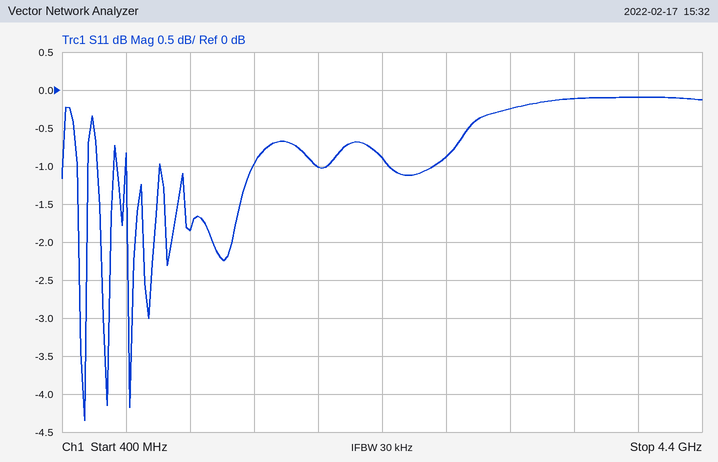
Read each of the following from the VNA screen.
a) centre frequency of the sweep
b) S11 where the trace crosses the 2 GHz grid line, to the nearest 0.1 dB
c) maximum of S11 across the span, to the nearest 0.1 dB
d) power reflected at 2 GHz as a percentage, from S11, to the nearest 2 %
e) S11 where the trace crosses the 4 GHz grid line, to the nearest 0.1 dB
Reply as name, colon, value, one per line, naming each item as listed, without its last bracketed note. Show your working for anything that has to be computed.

centre frequency of the sweep: 2.4 GHz
S11 where the trace crosses the 2 GHz grid line, to the nearest 0.1 dB: -1.0 dB
maximum of S11 across the span, to the nearest 0.1 dB: -0.1 dB
power reflected at 2 GHz as a percentage, from S11, to the nearest 2 %: 10^(-1/10) ≈ 79.4 %, so 80 % to the nearest 2 %
S11 where the trace crosses the 4 GHz grid line, to the nearest 0.1 dB: -0.1 dB
